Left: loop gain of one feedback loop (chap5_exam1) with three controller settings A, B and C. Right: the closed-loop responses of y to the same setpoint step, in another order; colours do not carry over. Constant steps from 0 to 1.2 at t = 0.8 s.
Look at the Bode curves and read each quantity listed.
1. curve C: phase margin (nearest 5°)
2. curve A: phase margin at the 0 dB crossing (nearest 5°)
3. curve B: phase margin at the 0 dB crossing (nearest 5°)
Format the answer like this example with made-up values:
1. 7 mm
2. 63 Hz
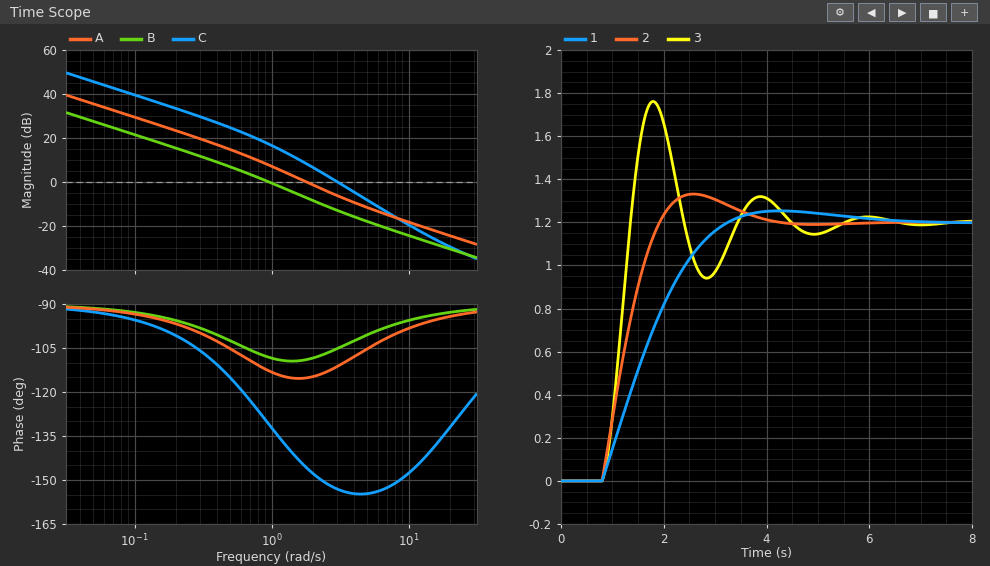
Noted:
1. 25°
2. 65°
3. 70°
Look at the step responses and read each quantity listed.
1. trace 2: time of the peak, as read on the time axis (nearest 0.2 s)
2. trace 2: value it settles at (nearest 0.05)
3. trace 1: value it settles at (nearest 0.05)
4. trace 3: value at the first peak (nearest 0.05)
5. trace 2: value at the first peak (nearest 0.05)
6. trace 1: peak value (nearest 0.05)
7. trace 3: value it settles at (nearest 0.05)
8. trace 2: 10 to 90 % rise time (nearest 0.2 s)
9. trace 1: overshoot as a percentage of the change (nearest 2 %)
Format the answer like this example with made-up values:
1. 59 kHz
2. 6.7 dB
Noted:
1. 2.6 s
2. 1.20
3. 1.20
4. 1.75
5. 1.35
6. 1.25
7. 1.20
8. 0.8 s
9. 4 %
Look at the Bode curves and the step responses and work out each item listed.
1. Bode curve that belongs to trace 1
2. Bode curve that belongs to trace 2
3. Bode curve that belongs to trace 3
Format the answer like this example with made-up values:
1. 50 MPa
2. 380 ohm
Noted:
1. B
2. A
3. C
